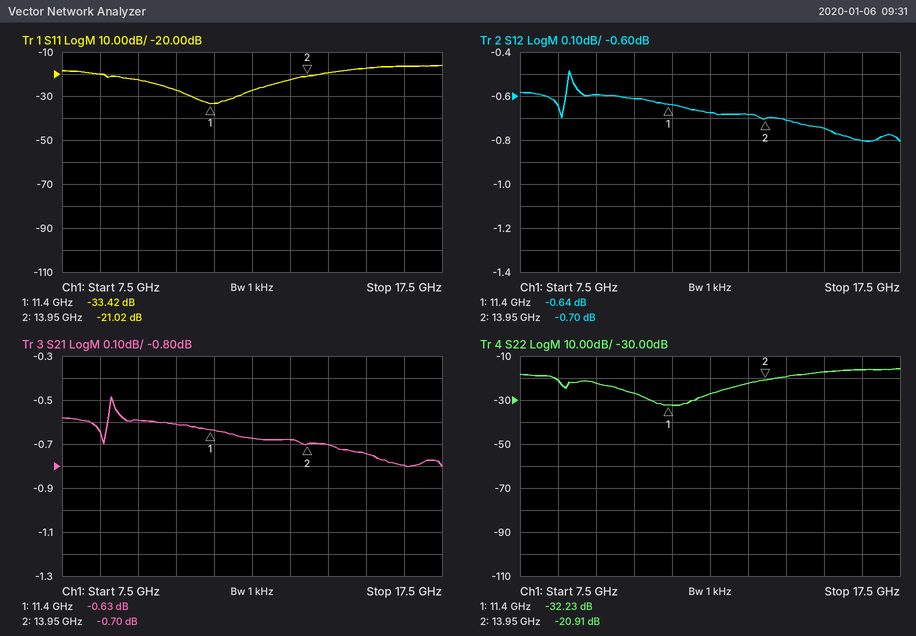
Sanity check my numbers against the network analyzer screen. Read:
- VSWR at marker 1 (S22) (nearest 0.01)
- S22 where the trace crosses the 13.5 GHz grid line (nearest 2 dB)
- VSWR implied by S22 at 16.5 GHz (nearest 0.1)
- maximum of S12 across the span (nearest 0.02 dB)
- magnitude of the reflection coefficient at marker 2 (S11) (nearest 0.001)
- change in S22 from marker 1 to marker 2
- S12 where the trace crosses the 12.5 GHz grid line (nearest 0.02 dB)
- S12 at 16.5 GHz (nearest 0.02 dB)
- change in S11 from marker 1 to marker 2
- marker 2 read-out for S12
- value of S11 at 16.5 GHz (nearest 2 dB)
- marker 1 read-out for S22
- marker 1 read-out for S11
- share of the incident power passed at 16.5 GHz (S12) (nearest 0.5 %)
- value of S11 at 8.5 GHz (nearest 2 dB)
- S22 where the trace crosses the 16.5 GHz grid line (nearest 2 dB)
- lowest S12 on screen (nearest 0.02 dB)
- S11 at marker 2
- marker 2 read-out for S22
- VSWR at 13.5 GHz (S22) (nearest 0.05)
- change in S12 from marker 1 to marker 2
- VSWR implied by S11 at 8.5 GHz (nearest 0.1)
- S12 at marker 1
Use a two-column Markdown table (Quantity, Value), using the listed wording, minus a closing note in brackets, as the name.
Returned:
| Quantity | Value |
|---|---|
| VSWR at marker 1 (S22) | 1.05 |
| S22 where the trace crosses the 13.5 GHz grid line | -22 dB |
| VSWR implied by S22 at 16.5 GHz | 1.4 |
| maximum of S12 across the span | -0.48 dB |
| magnitude of the reflection coefficient at marker 2 (S11) | 0.089 |
| change in S22 from marker 1 to marker 2 | 11.32 dB |
| S12 where the trace crosses the 12.5 GHz grid line | -0.68 dB |
| S12 at 16.5 GHz | -0.80 dB |
| change in S11 from marker 1 to marker 2 | 12.40 dB |
| marker 2 read-out for S12 | -0.70 dB |
| value of S11 at 16.5 GHz | -16 dB |
| marker 1 read-out for S22 | -32.23 dB |
| marker 1 read-out for S11 | -33.42 dB |
| share of the incident power passed at 16.5 GHz (S12) | 83.0 % |
| value of S11 at 8.5 GHz | -20 dB |
| S22 where the trace crosses the 16.5 GHz grid line | -16 dB |
| lowest S12 on screen | -0.80 dB |
| S11 at marker 2 | -21.02 dB |
| marker 2 read-out for S22 | -20.91 dB |
| VSWR at 13.5 GHz (S22) | 1.15 |
| change in S12 from marker 1 to marker 2 | -0.06 dB |
| VSWR implied by S11 at 8.5 GHz | 1.2 |
| S12 at marker 1 | -0.64 dB |
